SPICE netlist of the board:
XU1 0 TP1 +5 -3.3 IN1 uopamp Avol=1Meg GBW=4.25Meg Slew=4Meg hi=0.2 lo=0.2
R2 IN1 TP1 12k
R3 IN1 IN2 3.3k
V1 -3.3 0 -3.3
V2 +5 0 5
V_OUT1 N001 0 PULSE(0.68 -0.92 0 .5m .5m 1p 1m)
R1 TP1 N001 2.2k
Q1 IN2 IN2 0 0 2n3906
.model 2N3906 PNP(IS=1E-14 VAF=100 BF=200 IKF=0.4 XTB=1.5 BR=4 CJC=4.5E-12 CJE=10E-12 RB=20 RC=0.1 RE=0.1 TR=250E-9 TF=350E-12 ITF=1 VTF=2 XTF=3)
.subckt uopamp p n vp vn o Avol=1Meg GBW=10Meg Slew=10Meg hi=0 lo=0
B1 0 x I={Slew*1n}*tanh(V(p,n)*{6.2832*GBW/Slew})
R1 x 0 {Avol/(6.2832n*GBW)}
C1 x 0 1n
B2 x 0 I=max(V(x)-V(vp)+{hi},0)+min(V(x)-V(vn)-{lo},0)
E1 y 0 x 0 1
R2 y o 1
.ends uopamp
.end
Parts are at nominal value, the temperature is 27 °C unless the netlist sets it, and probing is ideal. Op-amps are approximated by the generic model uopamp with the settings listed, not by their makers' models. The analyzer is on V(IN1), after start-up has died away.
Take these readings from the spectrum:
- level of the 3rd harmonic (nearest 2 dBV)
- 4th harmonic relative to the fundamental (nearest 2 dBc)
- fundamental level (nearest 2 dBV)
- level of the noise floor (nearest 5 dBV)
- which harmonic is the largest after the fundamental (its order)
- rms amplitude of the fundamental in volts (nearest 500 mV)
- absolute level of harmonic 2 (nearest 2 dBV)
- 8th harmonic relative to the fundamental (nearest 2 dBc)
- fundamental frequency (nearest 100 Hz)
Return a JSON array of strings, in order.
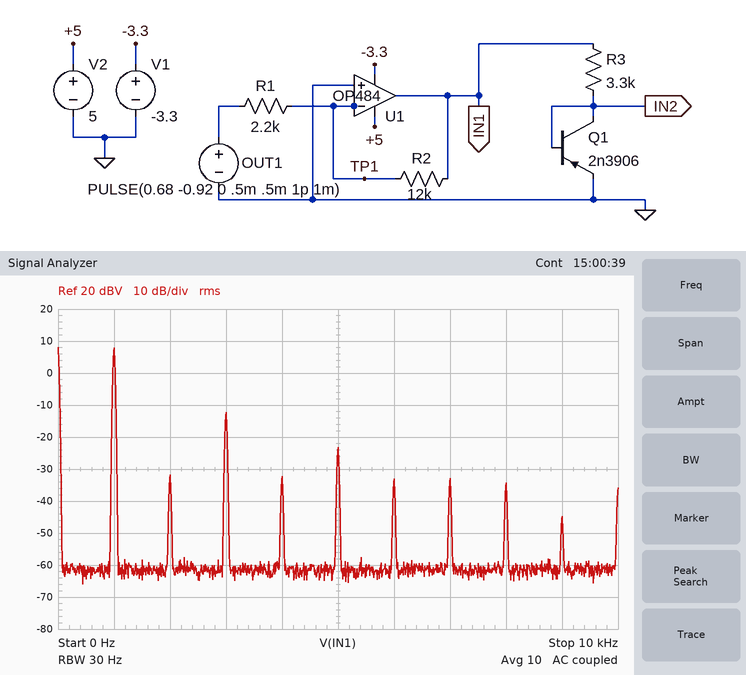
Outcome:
["-12 dBV", "-40 dBc", "8 dBV", "-60 dBV", "3", "2.5 V", "-32 dBV", "-42 dBc", "1.0 kHz"]
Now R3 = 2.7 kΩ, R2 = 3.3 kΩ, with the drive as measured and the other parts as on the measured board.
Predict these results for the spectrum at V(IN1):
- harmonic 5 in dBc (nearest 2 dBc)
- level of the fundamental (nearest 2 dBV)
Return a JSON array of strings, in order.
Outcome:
["-28 dBc", "-4 dBV"]
